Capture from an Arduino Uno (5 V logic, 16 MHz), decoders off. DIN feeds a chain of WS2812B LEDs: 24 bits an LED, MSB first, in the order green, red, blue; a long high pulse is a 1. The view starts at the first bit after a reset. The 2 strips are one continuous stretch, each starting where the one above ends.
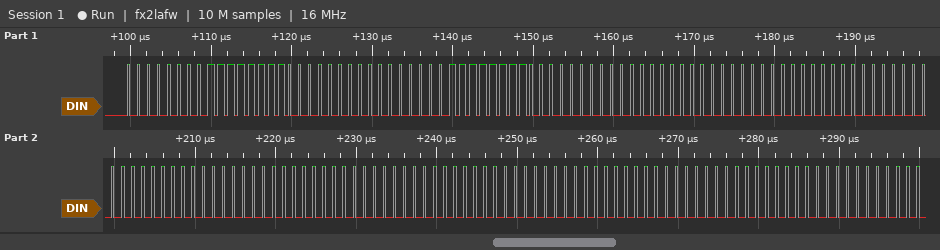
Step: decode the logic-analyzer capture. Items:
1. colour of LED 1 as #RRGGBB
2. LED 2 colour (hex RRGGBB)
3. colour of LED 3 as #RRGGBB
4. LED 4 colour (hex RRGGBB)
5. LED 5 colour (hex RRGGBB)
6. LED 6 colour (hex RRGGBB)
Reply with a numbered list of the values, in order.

1. #FF0000
2. #FF0000
3. #000000
4. #000000
5. #000000
6. #000000
